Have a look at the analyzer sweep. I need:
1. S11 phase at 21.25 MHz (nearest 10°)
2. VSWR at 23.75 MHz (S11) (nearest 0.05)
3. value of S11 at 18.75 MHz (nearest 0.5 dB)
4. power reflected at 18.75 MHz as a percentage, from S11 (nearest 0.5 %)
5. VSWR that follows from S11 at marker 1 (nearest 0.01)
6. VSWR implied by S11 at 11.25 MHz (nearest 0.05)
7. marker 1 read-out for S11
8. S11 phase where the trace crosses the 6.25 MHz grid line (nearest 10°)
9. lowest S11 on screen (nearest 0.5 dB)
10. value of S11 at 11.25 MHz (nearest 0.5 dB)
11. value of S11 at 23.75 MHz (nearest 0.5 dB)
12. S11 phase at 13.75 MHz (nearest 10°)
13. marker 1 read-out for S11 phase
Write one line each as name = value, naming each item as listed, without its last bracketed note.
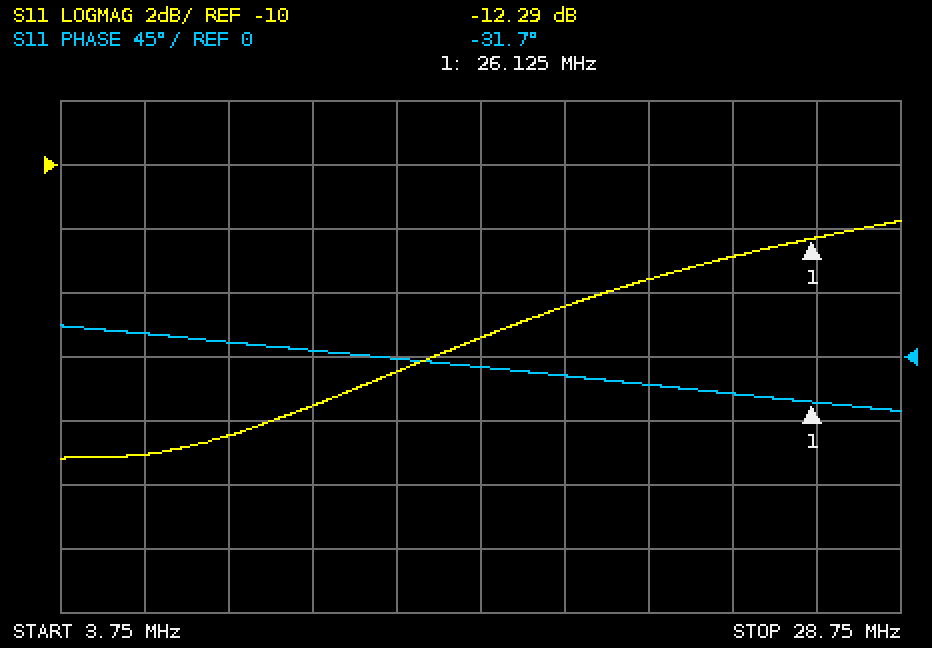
S11 phase at 21.25 MHz = -20°
VSWR at 23.75 MHz (S11) = 1.60
value of S11 at 18.75 MHz = -14.5 dB
power reflected at 18.75 MHz as a percentage, from S11 = 3.5 %
VSWR that follows from S11 at marker 1 = 1.64
VSWR implied by S11 at 11.25 MHz = 1.30
marker 1 read-out for S11 = -12.29 dB
S11 phase where the trace crosses the 6.25 MHz grid line = 20°
lowest S11 on screen = -19.0 dB
value of S11 at 11.25 MHz = -17.5 dB
value of S11 at 23.75 MHz = -13.0 dB
S11 phase at 13.75 MHz = 0°
marker 1 read-out for S11 phase = -31.7°
